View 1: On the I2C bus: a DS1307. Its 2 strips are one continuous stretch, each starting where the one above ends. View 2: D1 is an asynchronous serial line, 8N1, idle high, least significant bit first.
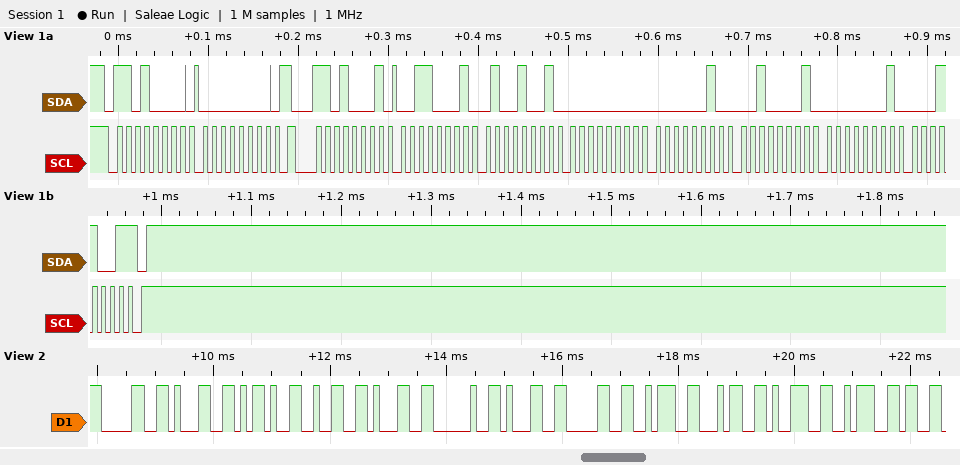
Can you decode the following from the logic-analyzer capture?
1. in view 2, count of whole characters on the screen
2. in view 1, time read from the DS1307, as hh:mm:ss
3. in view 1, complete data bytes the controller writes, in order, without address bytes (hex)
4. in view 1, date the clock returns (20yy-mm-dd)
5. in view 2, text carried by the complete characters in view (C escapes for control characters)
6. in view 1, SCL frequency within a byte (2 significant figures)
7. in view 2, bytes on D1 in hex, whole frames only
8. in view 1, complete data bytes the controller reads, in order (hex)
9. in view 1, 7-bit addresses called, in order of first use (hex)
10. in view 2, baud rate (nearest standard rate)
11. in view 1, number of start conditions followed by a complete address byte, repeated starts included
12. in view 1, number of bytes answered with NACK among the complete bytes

12
00:49:31
00
2019-01-21
"01-21 10:49:"
100 kHz
30 31 2D 32 31 20 31 30 3A 34 39 3A
31 49 00 02 21 01 19
0x68
9600 baud
2
1
